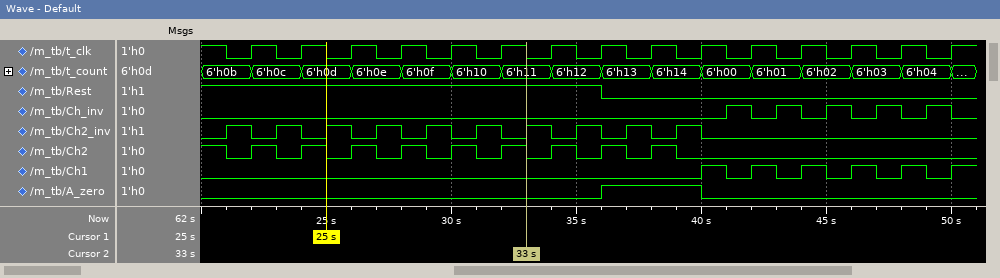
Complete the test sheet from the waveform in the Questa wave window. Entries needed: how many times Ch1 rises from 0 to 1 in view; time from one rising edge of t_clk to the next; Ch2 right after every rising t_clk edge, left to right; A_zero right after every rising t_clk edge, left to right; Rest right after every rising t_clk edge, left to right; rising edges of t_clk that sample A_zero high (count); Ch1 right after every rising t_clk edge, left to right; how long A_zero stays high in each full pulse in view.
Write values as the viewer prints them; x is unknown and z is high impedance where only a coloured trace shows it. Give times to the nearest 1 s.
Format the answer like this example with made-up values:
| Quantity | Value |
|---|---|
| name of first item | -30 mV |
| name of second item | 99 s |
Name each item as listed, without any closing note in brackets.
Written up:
| Quantity | Value |
|---|---|
| how many times Ch1 rises from 0 to 1 in view | 6 |
| time from one rising edge of t_clk to the next | 2 s |
| Ch2 right after every rising t_clk edge, left to right | 1 1 1 1 1 1 1 1 1 0 0 0 0 0 0 |
| A_zero right after every rising t_clk edge, left to right | 0 0 0 0 0 0 0 1 1 0 0 0 0 0 0 |
| Rest right after every rising t_clk edge, left to right | 1 1 1 1 1 1 1 0 0 0 0 0 0 0 0 |
| rising edges of t_clk that sample A_zero high | 2 |
| Ch1 right after every rising t_clk edge, left to right | 0 0 0 0 0 0 0 0 0 1 1 1 1 1 1 |
| how long A_zero stays high in each full pulse in view | 4 s |
